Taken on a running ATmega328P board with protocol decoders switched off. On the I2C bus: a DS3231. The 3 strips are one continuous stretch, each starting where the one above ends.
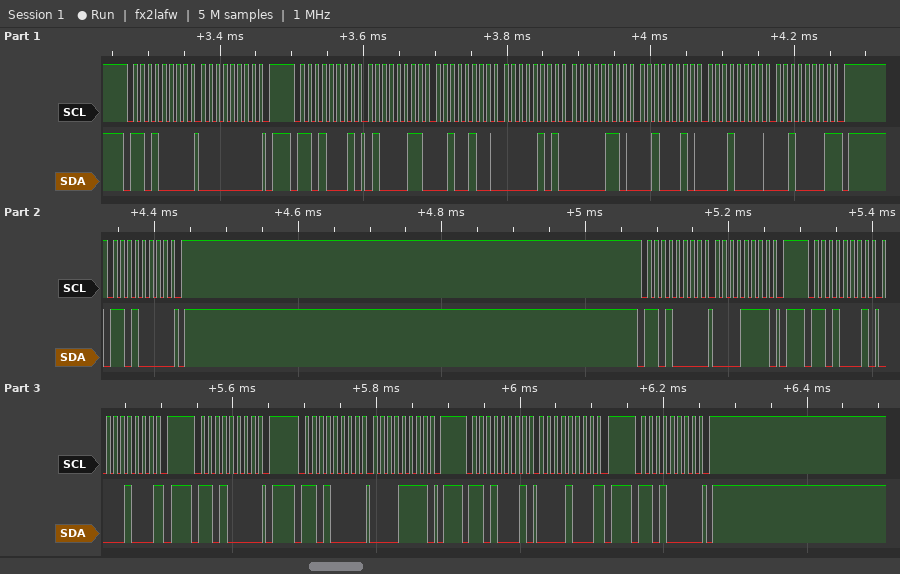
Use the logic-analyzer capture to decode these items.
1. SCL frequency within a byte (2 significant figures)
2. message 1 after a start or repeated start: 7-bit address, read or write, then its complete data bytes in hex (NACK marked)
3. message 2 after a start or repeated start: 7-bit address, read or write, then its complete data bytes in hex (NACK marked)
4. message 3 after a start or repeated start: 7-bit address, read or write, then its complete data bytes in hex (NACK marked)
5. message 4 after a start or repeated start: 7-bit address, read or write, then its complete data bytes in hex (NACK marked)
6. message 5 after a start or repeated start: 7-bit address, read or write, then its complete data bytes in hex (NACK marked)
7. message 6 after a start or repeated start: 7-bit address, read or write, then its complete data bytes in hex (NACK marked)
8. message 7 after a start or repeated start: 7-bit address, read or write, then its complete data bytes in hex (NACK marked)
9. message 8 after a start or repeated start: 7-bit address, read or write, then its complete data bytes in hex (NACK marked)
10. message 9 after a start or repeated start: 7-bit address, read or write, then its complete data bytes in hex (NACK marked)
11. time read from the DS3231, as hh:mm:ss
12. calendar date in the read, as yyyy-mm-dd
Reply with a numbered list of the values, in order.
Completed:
1. 100 kHz
2. 0x68 write: 00
3. 0x68 read: 43 24 05 06 22 10 21 NACK
4. 0x68 write
5. 0x68 write: 0F
6. 0x68 read: 08 NACK
7. 0x68 write
8. 0x68 write: 0F
9. 0x68 read: 08 NACK
10. 0x68 write
11. 05:24:43
12. 2021-10-22
